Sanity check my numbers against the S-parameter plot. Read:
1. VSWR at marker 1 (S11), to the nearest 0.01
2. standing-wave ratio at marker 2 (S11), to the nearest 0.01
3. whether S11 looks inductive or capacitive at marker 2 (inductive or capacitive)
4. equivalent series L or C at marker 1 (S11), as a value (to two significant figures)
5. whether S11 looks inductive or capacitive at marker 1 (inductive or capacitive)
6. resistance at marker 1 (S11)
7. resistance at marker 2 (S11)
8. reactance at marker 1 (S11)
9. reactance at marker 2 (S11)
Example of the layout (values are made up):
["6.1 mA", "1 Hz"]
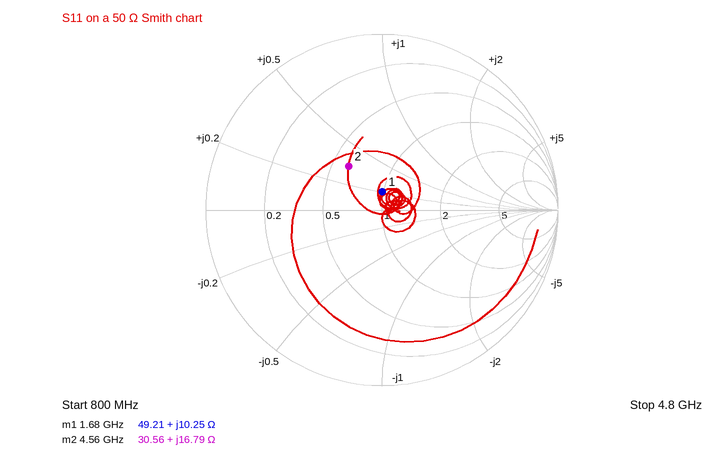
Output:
["1.23", "1.91", "inductive", "970 pH", "inductive", "49.21 Ω", "30.56 Ω", "+10.25 Ω", "+16.79 Ω"]
